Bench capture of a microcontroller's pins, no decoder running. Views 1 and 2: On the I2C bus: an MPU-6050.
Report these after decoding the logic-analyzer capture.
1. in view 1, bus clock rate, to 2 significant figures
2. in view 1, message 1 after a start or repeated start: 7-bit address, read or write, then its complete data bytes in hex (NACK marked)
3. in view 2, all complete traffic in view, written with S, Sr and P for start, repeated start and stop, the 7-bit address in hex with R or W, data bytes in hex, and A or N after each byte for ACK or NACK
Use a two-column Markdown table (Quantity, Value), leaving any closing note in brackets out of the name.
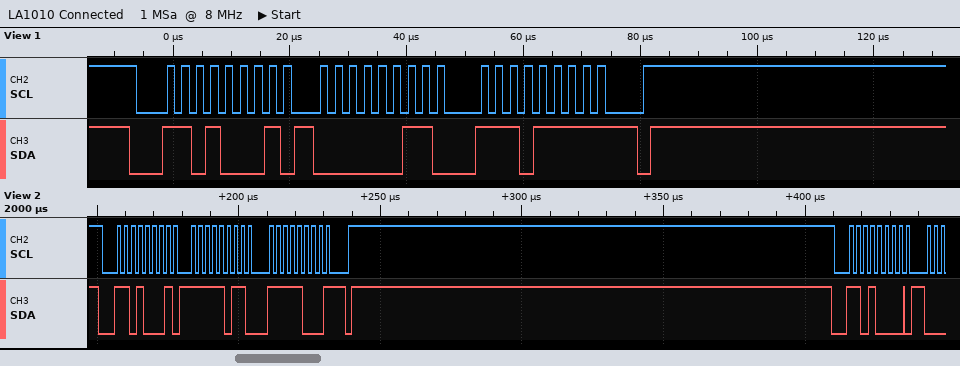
| Quantity | Value |
|---|---|
| in view 1, bus clock rate, to 2 significant figures | 400 kHz |
| in view 1, message 1 after a start or repeated start: 7-bit address, read or write, then its complete data bytes in hex | 0x68 read: 03 EF NACK |
| in view 2, all complete traffic in view, written with S, Sr and P for start, repeated start and stop, the 7-bit address in hex with R or W, data bytes in hex, and A or N after each byte for ACK or NACK | S 68R A FB A F8 N P S 68W A |
